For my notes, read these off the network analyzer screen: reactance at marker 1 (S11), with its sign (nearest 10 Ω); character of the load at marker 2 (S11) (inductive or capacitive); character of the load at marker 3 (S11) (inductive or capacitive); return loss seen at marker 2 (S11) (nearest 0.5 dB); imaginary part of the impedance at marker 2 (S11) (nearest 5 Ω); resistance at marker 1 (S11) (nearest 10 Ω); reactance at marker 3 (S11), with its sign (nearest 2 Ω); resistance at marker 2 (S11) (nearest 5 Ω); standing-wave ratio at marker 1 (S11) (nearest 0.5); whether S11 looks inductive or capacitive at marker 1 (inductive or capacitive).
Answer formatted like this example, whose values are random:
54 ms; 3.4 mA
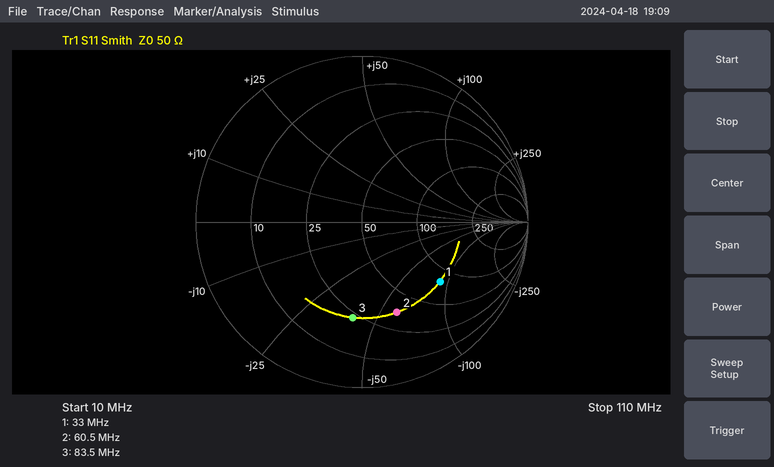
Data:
-90 Ω; capacitive; capacitive; 4.5 dB; -60 Ω; 80 Ω; -40 Ω; 35 Ω; 4.0; capacitive
